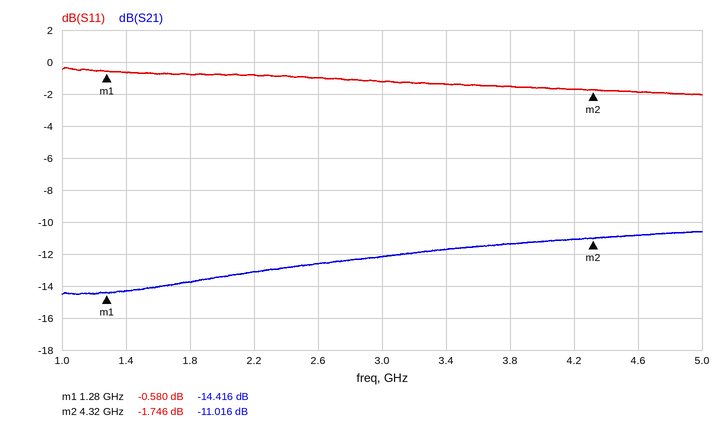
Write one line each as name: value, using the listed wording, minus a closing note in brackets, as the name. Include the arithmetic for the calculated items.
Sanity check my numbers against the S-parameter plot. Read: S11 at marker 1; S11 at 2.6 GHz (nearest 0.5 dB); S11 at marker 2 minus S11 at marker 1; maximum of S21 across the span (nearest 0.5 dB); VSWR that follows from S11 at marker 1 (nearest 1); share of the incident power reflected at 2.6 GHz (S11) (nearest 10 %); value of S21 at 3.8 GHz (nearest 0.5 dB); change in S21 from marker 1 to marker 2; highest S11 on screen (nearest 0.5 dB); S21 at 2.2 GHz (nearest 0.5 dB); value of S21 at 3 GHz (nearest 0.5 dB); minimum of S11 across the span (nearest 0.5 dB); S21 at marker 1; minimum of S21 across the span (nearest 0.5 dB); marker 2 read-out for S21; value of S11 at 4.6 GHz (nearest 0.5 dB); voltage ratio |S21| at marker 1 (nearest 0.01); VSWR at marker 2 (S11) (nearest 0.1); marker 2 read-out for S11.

S11 at marker 1: -0.580 dB
S11 at 2.6 GHz: -1.0 dB
S11 at marker 2 minus S11 at marker 1: -1.746 − (-0.58) = -1.166 dB
maximum of S21 across the span: -10.5 dB
VSWR that follows from S11 at marker 1: (1 + 0.9354)/(1 − 0.9354) ≈ 30
share of the incident power reflected at 2.6 GHz (S11): 10^(-1/10) ≈ 79.4 %, so 80 % to the nearest 10 %
value of S21 at 3.8 GHz: -11.5 dB
change in S21 from marker 1 to marker 2: -11.016 − (-14.416) = 3.400 dB
highest S11 on screen: -0.5 dB
S21 at 2.2 GHz: -13.0 dB
value of S21 at 3 GHz: -12.0 dB
minimum of S11 across the span: -2.0 dB
S21 at marker 1: -14.416 dB
minimum of S21 across the span: -14.5 dB
marker 2 read-out for S21: -11.016 dB
value of S11 at 4.6 GHz: -2.0 dB
voltage ratio |S21| at marker 1: 10^(-14.416/20) ≈ 0.19
VSWR at marker 2 (S11): (1 + 0.8179)/(1 − 0.8179) ≈ 10.0
marker 2 read-out for S11: -1.746 dB
